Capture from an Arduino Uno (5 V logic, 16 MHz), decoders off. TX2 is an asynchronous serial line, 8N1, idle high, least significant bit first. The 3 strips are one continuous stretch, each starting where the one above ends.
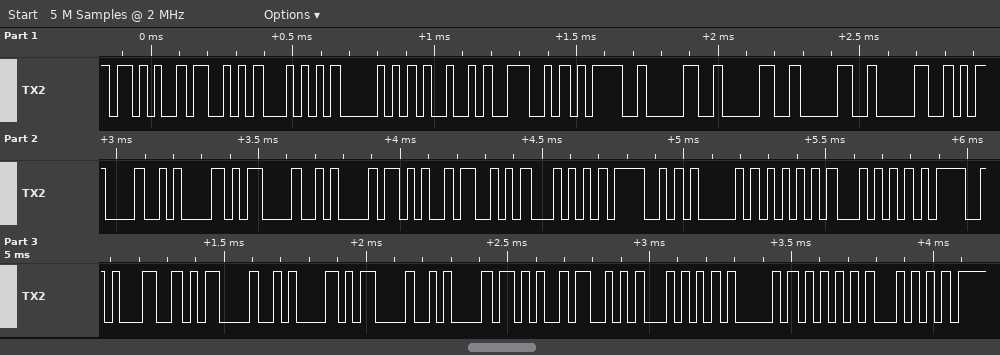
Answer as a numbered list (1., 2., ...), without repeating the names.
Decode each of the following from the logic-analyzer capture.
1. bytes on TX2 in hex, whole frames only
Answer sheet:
1. 0x2B 0x53 0x54 0x50 0x49 0x4E 0x3D 0x30 0x30 0x30 0x30 0x0D 0x0A 0x0D 0x0A 0x2B 0x53 0x54 0x4F 0x41 0x55 0x54 0x3D 0x31 0x0D 0x0A 0x0D 0x0A 0x2B 0x53 0x54 0x41 0x55 0x54
